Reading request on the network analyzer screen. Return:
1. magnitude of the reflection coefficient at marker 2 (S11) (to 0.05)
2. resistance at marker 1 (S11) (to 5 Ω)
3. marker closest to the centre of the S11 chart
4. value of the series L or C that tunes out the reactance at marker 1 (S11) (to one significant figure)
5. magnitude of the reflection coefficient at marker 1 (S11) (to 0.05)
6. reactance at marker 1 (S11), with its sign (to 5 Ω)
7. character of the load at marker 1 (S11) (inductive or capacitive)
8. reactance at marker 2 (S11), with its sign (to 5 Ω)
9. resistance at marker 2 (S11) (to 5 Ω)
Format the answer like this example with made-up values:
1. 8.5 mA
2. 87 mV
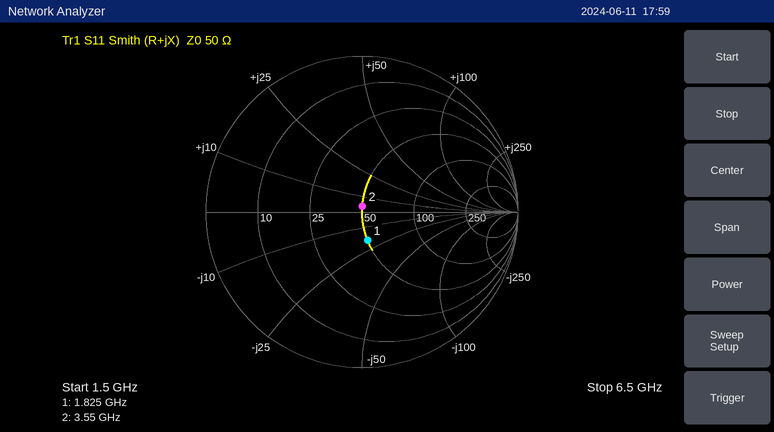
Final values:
1. 0.05
2. 50 Ω
3. marker 2
4. 2 nH
5. 0.20
6. -20 Ω
7. capacitive
8. +5 Ω
9. 50 Ω
